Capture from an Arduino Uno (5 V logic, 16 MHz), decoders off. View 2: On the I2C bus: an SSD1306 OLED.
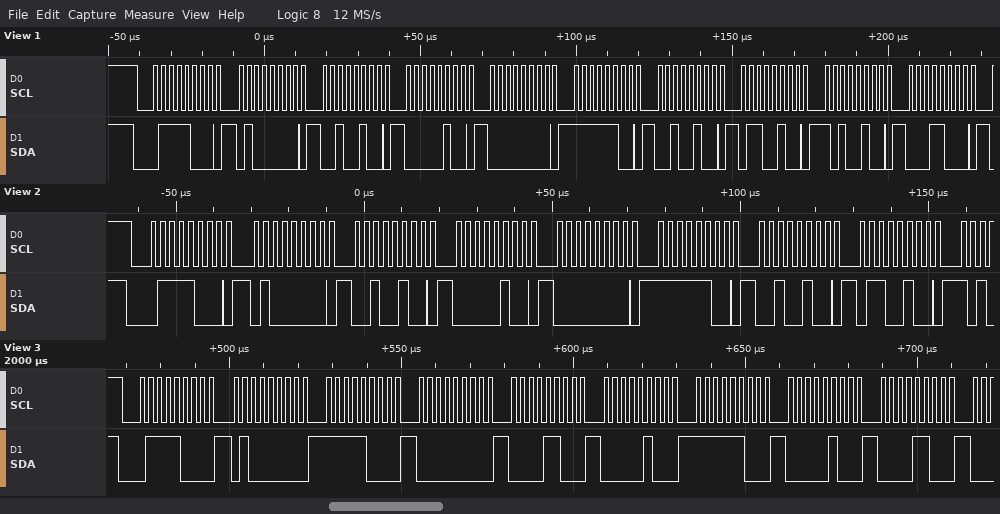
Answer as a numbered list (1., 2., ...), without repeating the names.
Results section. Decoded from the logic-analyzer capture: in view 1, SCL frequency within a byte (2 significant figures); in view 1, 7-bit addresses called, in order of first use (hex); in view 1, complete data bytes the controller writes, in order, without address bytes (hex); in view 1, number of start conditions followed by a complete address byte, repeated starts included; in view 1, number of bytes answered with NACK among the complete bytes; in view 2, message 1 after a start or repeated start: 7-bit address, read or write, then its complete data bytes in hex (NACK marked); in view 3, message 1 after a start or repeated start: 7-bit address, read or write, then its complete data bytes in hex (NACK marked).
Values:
1. 400 kHz
2. 0x3C
3. 40 24 04 00 FC 24 64 A4 18
4. 1
5. 0
6. 0x3C write: 40 24 04 00 FC 24 64
7. 0x3C write: 40 F8 00 0C 04 FC 04 0C
